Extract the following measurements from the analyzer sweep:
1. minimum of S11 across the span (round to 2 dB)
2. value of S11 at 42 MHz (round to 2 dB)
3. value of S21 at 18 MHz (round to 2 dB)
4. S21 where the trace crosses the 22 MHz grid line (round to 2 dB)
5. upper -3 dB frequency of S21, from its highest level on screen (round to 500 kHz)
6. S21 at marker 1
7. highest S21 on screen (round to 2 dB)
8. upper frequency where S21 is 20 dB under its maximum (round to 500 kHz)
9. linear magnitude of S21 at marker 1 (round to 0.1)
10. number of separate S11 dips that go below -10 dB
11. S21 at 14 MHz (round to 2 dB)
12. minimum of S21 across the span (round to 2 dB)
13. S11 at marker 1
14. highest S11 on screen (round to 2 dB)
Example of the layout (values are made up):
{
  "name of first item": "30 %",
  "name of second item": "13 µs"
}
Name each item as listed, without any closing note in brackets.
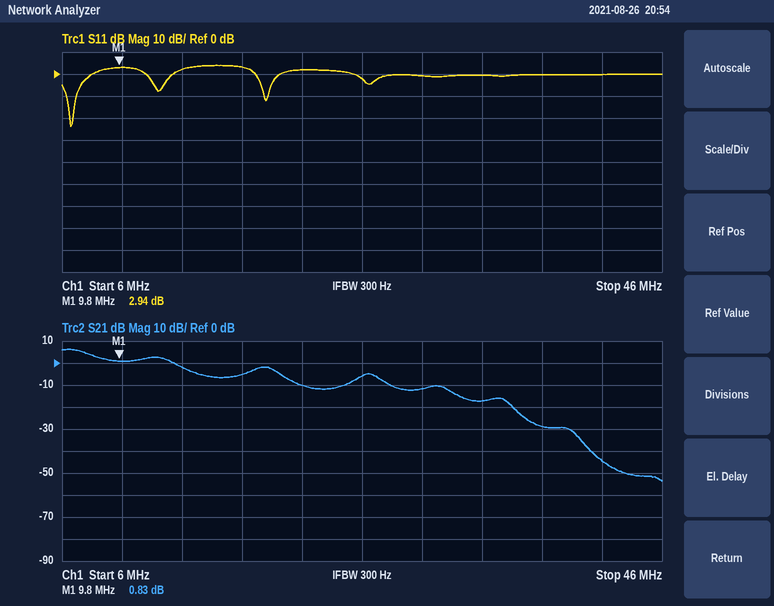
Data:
{
  "minimum of S11 across the span": "-24 dB",
  "value of S11 at 42 MHz": "0 dB",
  "value of S21 at 18 MHz": "-6 dB",
  "S21 where the trace crosses the 22 MHz grid line": "-10 dB",
  "upper -3 dB frequency of S21, from its highest level on screen": "8.0 MHz",
  "S21 at marker 1": "0.83 dB",
  "highest S21 on screen": "6 dB",
  "upper frequency where S21 is 20 dB under its maximum": "32.0 MHz",
  "linear magnitude of S21 at marker 1": "1.1",
  "number of separate S11 dips that go below -10 dB": "2",
  "S21 at 14 MHz": "-2 dB",
  "minimum of S21 across the span": "-54 dB",
  "S11 at marker 1": "2.94 dB",
  "highest S11 on screen": "4 dB"
}
